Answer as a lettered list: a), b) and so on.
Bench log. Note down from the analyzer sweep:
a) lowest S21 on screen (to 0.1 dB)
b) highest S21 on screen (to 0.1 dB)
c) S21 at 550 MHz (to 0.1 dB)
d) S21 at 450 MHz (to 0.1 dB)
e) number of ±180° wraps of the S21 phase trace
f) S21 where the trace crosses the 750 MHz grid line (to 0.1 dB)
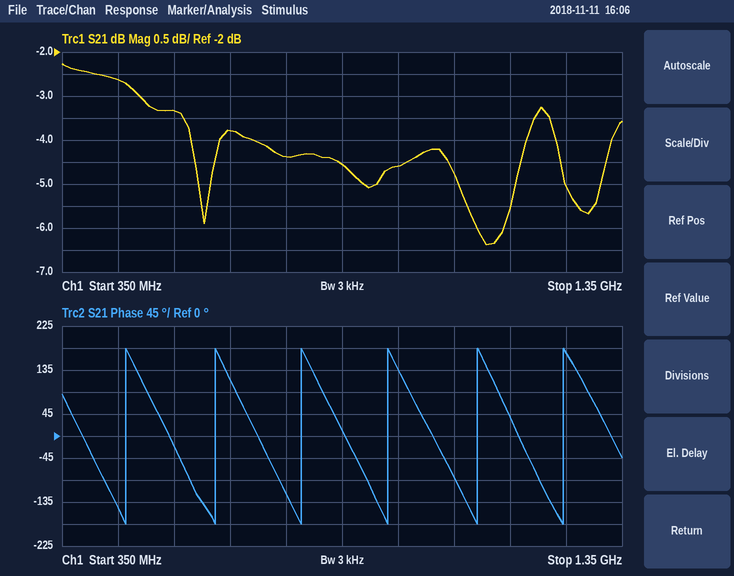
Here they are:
a) -6.4 dB
b) -2.3 dB
c) -3.3 dB
d) -2.6 dB
e) 6
f) -4.4 dB
